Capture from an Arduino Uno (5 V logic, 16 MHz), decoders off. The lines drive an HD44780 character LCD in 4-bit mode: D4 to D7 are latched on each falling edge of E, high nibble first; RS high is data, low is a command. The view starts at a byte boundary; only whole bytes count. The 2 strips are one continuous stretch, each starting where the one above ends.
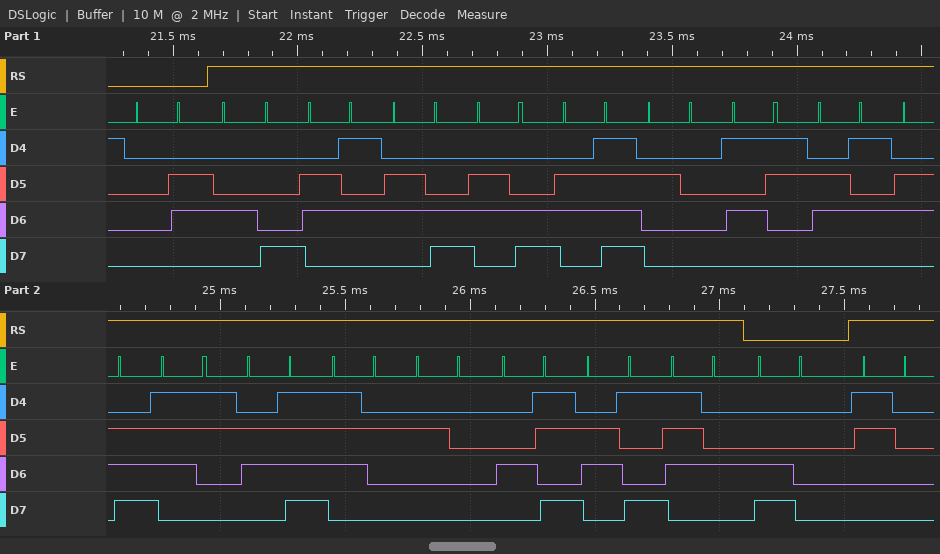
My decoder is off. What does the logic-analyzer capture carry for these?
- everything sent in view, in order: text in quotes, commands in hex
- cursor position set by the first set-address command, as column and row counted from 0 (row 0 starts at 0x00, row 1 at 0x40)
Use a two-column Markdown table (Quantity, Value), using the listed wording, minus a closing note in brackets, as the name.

| Quantity | Value |
|---|---|
| everything sent in view, in order: text in quotes, commands in hex | 0x06 "Hello Sensor Kit" 0xC0 "0" |
| cursor position set by the first set-address command, as column and row counted from 0 | column 0, row 1 |
